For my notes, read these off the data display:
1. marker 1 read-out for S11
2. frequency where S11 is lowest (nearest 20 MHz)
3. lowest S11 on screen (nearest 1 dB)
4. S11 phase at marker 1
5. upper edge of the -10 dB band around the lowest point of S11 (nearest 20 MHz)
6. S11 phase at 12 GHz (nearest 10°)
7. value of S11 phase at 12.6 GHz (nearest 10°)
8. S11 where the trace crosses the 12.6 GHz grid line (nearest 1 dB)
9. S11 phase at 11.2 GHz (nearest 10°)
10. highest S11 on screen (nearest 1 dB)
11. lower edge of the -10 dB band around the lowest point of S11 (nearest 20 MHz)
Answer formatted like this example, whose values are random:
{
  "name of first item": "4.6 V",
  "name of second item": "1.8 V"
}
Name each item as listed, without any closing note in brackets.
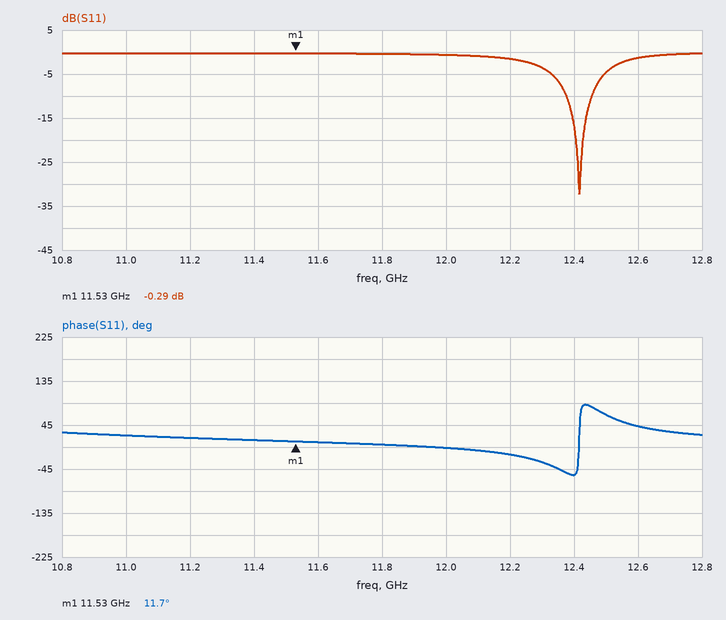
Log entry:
{
  "marker 1 read-out for S11": "-0.29 dB",
  "frequency where S11 is lowest": "12.42 GHz",
  "lowest S11 on screen": "-32 dB",
  "S11 phase at marker 1": "11.7°",
  "upper edge of the -10 dB band around the lowest point of S11": "12.46 GHz",
  "S11 phase at 12 GHz": "0°",
  "value of S11 phase at 12.6 GHz": "40°",
  "S11 where the trace crosses the 12.6 GHz grid line": "-1 dB",
  "S11 phase at 11.2 GHz": "20°",
  "highest S11 on screen": "0 dB",
  "lower edge of the -10 dB band around the lowest point of S11": "12.38 GHz"
}
